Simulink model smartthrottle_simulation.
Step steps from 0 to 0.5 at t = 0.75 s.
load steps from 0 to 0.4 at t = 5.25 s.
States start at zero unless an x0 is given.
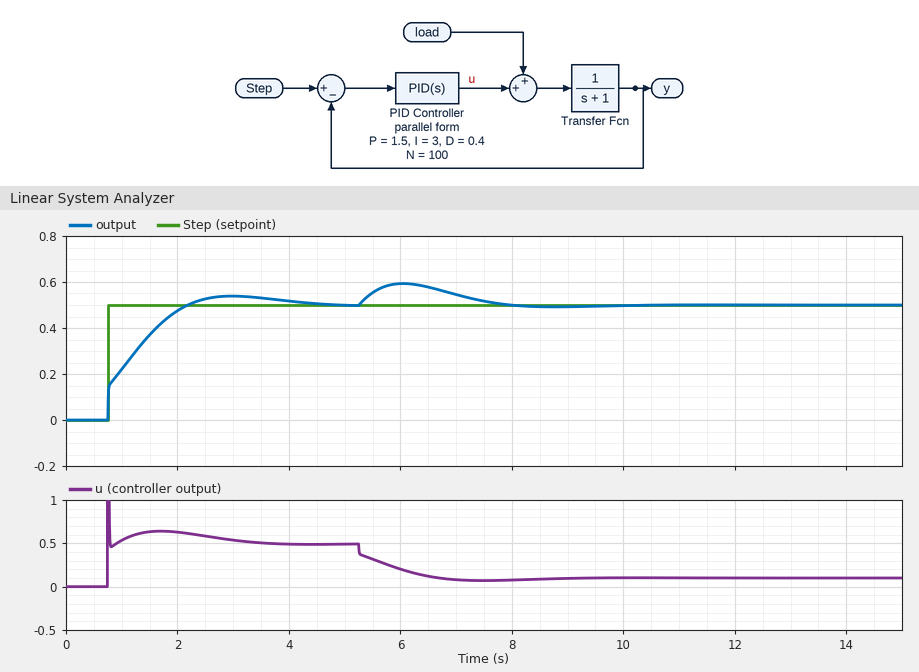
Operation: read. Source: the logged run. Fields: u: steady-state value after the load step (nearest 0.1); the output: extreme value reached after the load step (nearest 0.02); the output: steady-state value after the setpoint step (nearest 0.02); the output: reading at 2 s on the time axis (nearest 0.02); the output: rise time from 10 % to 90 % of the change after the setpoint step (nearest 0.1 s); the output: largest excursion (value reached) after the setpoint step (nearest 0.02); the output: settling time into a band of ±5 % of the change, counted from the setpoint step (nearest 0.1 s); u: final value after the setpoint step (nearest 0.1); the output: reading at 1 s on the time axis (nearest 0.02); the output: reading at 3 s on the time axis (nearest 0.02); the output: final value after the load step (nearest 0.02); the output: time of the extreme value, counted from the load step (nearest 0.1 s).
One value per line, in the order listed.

0.1
0.60
0.50
0.48
1.1 s
0.54
3.0 s
0.5
0.22
0.54
0.50
0.8 s
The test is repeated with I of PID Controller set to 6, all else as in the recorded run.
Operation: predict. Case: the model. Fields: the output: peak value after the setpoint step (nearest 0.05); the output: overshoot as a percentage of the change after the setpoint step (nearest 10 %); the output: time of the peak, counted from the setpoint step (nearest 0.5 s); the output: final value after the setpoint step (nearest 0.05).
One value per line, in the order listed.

0.60
20 %
1.5 s
0.50
